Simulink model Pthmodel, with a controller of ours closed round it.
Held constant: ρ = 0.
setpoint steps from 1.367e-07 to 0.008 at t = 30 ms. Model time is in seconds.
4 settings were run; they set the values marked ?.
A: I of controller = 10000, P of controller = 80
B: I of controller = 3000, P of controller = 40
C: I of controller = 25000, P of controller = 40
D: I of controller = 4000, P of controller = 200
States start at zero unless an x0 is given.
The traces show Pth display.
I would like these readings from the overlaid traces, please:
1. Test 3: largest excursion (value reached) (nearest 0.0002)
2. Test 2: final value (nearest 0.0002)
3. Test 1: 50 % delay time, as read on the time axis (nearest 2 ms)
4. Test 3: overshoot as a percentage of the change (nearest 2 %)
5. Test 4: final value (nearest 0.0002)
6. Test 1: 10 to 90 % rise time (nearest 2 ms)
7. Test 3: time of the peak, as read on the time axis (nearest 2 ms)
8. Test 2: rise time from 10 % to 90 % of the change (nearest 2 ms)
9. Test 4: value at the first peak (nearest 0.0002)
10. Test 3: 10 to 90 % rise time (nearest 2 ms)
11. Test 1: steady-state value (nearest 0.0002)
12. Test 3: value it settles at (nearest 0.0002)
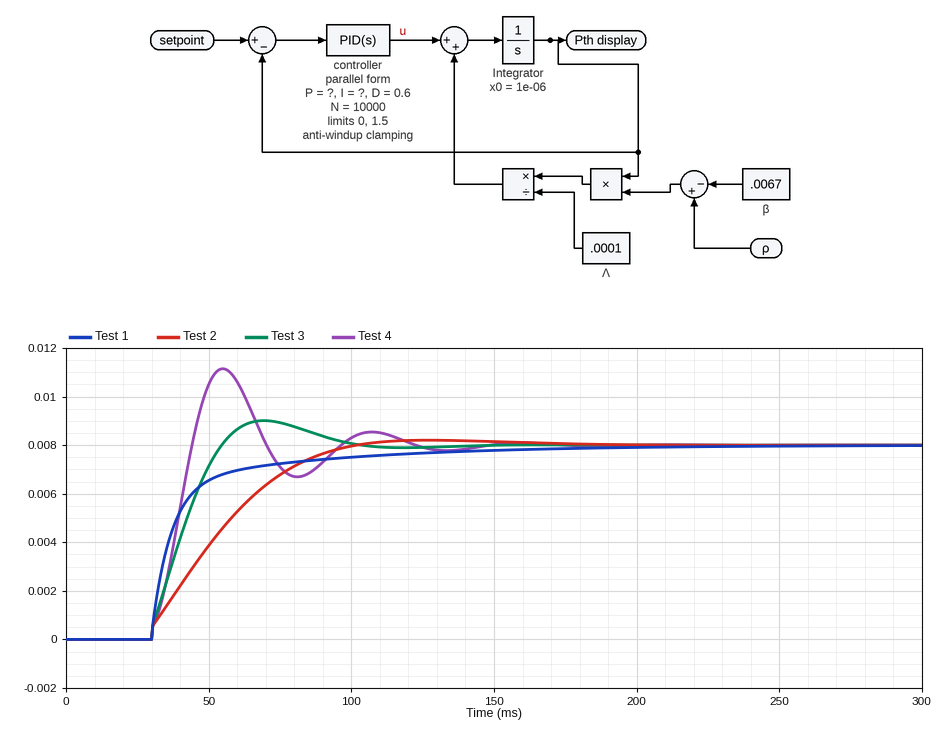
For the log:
0.0090
0.0080
36 ms
12 %
0.0080
42 ms
70 ms
50 ms
0.0112
20 ms
0.0080
0.0080
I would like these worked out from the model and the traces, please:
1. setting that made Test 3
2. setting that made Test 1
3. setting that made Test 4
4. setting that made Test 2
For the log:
A
D
C
B
